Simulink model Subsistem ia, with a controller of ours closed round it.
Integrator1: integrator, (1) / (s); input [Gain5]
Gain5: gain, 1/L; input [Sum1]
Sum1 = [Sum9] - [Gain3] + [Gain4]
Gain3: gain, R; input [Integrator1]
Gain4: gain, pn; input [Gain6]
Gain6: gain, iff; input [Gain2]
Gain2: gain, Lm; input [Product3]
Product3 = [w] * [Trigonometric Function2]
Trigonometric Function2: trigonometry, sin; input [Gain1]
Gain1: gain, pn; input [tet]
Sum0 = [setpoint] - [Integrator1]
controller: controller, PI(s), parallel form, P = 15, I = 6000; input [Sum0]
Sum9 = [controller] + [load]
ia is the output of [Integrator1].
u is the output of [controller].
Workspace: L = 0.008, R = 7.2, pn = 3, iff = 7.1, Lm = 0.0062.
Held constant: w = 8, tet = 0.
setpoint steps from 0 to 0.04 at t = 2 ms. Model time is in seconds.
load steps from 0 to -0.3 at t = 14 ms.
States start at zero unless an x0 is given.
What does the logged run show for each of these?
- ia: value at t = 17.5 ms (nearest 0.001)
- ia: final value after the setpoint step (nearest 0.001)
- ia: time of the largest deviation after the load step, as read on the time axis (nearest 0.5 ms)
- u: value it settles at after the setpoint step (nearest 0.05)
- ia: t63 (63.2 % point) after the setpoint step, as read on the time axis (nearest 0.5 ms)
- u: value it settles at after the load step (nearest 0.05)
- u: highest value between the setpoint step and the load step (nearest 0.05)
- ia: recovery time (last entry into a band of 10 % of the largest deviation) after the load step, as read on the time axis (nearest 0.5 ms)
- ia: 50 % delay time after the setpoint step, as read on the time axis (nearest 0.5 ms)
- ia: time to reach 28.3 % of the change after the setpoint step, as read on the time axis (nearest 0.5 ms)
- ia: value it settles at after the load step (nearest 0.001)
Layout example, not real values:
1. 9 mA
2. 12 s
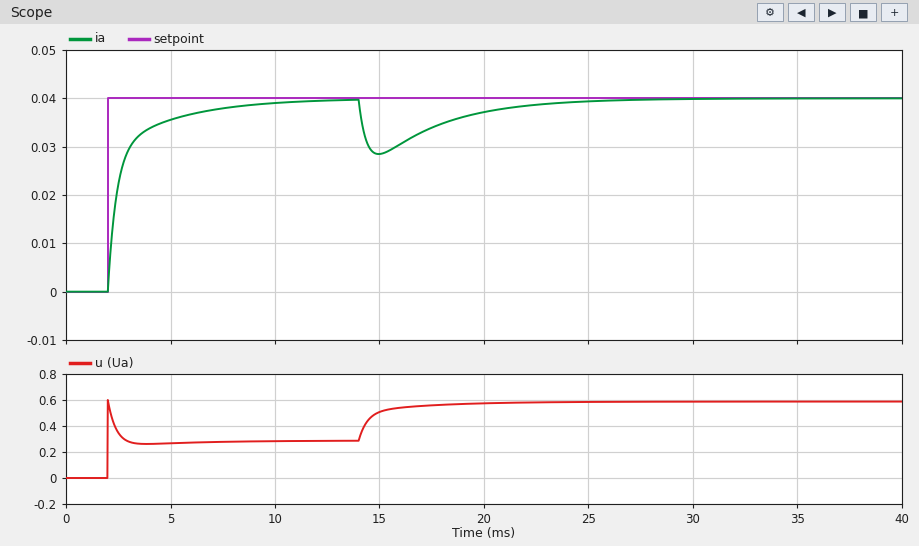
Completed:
1. 0.034
2. 0.040
3. 15.0 ms
4. 0.30
5. 2.5 ms
6. 0.60
7. 0.60
8. 23.0 ms
9. 2.5 ms
10. 2.0 ms
11. 0.040
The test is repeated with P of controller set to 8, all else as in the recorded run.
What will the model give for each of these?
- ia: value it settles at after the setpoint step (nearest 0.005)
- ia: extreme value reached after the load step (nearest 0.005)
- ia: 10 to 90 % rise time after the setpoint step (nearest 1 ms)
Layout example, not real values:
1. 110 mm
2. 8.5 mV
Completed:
1. 0.040
2. 0.025
3. 3 ms
